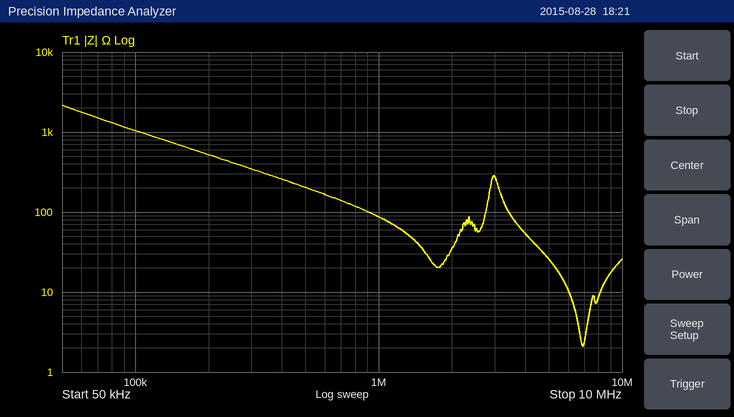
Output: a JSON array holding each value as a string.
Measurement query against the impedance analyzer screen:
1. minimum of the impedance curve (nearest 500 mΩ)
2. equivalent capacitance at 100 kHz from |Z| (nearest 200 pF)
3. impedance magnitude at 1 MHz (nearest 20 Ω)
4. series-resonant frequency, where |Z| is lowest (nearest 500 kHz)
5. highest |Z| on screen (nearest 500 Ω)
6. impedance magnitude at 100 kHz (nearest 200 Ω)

["2.0 Ω", "1.6 nF", "80 Ω", "7.0 MHz", "2.0 kΩ", "1.0 kΩ"]
